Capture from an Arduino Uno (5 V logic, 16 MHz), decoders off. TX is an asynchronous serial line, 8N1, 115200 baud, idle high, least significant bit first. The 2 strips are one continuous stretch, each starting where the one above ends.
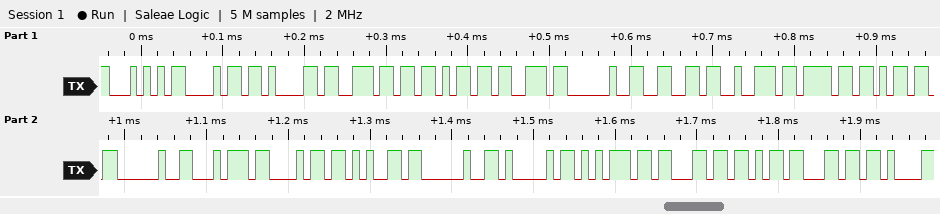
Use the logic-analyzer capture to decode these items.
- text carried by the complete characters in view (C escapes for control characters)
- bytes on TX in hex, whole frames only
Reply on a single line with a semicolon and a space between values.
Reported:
"Thanks from the Auckl"; 54 68 61 6E 6B 73 20 66 72 6F 6D 20 74 68 65 20 41 75 63 6B 6C
